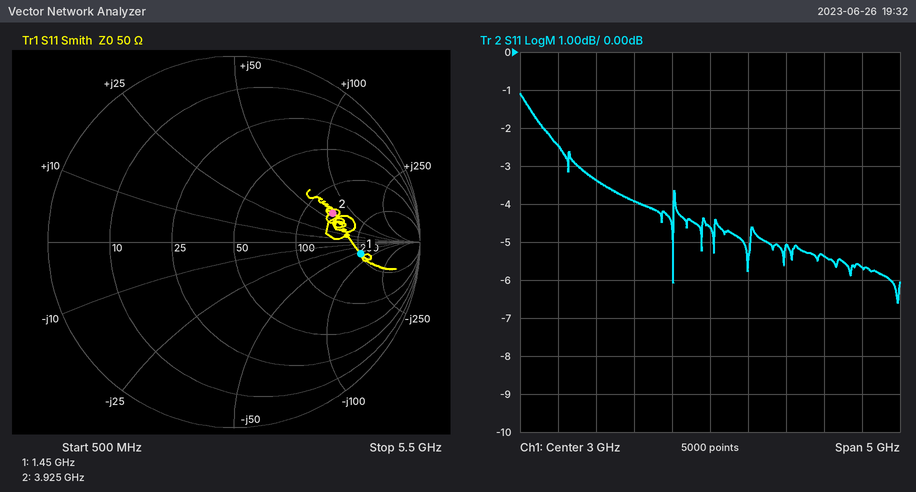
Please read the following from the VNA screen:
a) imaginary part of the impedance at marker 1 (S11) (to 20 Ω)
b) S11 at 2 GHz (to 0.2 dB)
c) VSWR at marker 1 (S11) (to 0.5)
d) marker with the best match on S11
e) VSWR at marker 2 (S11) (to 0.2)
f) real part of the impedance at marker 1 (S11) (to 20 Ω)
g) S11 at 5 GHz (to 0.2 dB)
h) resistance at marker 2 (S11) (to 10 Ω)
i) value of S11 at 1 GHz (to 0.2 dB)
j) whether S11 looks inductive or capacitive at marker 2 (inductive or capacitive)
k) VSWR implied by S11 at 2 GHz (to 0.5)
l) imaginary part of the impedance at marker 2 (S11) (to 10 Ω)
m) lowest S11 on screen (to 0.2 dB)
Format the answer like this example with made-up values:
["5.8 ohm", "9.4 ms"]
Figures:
["-60 Ω", "-4.0 dB", "5.5", "marker 2", "3.4", "260 Ω", "-5.6 dB", "140 Ω", "-2.4 dB", "inductive", "4.5", "+60 Ω", "-6.6 dB"]
